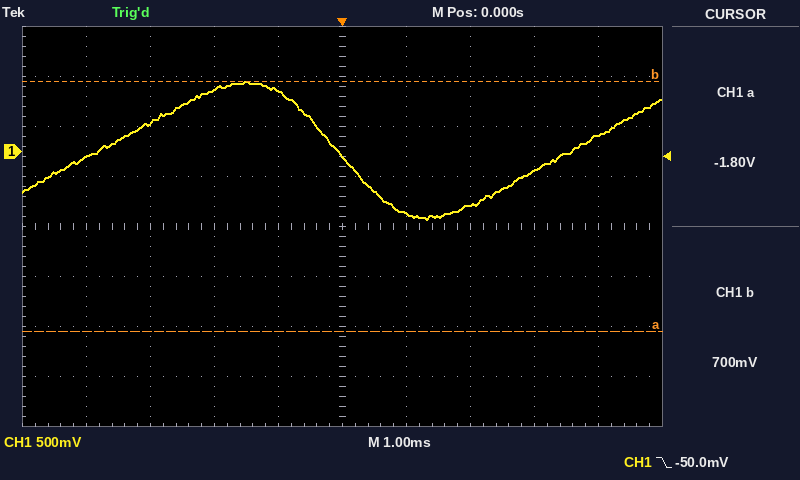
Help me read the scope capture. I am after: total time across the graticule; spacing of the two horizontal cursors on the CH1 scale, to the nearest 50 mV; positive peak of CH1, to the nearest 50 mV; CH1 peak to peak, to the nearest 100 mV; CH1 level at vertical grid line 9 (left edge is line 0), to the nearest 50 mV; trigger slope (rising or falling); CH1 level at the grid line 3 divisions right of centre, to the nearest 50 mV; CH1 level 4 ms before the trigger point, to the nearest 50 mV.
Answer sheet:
10 ms
2.50 V
700 mV
1.40 V
150 mV
falling
-200 mV
-50 mV
